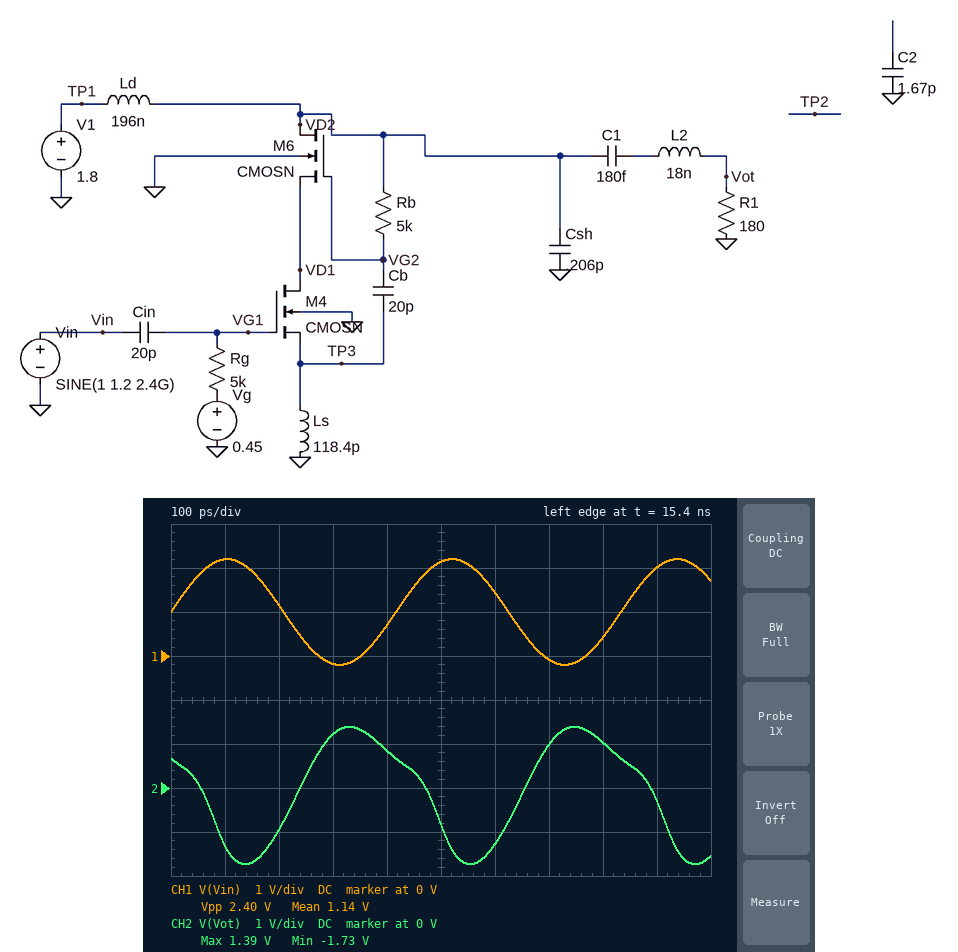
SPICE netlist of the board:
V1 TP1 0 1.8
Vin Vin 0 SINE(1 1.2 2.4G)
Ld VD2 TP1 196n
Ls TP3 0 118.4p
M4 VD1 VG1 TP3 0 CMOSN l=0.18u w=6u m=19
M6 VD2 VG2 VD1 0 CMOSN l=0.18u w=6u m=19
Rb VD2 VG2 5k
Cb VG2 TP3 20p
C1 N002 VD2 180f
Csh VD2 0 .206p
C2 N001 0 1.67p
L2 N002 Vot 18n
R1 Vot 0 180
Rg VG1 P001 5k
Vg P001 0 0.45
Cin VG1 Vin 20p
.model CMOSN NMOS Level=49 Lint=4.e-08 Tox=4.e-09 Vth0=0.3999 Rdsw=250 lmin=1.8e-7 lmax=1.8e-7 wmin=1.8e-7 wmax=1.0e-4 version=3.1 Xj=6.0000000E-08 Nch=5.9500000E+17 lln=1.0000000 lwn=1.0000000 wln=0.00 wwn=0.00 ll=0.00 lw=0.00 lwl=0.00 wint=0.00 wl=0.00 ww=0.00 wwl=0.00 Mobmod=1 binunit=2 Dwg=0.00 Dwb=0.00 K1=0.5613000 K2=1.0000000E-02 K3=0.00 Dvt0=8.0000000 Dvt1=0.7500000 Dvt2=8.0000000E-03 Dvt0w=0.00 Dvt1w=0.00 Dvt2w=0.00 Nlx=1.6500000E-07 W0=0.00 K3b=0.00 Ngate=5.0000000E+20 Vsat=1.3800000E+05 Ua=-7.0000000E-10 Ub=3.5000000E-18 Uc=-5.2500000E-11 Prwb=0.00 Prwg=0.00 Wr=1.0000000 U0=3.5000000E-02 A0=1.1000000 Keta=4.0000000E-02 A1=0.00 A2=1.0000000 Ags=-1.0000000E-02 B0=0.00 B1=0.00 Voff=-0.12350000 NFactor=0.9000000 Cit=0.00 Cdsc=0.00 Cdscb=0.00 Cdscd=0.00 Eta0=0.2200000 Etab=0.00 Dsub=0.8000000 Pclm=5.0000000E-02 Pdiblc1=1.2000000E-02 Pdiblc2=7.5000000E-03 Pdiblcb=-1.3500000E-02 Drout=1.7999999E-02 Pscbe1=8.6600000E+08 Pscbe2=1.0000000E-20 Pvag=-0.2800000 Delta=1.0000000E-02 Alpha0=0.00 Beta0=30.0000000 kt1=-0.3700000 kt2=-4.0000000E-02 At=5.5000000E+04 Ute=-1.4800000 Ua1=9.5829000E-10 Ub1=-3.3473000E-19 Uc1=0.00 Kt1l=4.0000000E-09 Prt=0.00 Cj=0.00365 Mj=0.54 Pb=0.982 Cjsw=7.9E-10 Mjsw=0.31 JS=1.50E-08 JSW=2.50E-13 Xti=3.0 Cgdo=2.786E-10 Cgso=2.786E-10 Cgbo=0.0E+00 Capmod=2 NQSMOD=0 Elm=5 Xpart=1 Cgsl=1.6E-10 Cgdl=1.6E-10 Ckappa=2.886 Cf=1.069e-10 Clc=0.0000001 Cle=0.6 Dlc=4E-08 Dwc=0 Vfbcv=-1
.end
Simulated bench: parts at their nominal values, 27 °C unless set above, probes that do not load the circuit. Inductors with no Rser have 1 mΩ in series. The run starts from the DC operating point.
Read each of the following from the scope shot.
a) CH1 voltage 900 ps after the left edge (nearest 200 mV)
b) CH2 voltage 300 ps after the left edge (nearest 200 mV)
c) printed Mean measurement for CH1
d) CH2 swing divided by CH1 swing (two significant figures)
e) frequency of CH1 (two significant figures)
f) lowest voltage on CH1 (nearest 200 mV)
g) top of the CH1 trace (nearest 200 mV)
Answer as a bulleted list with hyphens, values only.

- 2.0 V
- 1.2 V
- 1.14 V
- 1.3
- 2.4 GHz
- -200 mV
- 2.2 V
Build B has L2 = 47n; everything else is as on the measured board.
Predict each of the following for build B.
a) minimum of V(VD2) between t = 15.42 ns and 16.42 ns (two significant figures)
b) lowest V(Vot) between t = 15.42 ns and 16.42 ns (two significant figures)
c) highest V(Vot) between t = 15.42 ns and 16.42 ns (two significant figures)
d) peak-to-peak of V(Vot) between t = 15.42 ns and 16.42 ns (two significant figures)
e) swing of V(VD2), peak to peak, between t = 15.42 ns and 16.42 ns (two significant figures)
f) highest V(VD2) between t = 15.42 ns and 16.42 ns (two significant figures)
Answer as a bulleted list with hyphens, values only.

- -170 mV
- -960 mV
- 1.1 V
- 2.1 V
- 4.4 V
- 4.2 V
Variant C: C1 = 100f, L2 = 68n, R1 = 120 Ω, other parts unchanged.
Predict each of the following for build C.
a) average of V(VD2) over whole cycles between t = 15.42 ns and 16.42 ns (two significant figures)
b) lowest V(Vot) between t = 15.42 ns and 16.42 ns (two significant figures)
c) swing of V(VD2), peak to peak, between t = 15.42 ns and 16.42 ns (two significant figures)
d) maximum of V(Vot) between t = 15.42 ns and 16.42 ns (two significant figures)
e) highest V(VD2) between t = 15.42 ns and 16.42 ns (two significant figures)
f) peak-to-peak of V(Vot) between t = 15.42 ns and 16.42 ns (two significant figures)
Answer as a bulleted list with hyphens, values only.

- 1.8 V
- -670 mV
- 4.5 V
- 770 mV
- 4.3 V
- 1.4 V
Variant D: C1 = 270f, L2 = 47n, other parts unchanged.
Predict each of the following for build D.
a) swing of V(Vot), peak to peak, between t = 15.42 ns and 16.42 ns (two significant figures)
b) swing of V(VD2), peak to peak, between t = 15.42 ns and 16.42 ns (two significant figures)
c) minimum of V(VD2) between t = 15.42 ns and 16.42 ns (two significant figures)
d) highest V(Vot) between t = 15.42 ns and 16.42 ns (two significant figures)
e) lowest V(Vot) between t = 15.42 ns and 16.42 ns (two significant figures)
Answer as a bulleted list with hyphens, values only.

- 1.7 V
- 4.7 V
- -170 mV
- 950 mV
- -740 mV
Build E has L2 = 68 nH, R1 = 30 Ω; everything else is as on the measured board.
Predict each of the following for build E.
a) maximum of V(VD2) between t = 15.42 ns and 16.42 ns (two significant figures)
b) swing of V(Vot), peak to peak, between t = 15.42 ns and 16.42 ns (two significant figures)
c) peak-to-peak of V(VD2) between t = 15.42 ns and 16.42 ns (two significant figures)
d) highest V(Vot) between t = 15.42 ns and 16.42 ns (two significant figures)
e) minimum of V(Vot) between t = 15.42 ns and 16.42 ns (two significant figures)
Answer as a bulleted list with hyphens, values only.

- 4.9 V
- 220 mV
- 5.1 V
- 120 mV
- -98 mV
